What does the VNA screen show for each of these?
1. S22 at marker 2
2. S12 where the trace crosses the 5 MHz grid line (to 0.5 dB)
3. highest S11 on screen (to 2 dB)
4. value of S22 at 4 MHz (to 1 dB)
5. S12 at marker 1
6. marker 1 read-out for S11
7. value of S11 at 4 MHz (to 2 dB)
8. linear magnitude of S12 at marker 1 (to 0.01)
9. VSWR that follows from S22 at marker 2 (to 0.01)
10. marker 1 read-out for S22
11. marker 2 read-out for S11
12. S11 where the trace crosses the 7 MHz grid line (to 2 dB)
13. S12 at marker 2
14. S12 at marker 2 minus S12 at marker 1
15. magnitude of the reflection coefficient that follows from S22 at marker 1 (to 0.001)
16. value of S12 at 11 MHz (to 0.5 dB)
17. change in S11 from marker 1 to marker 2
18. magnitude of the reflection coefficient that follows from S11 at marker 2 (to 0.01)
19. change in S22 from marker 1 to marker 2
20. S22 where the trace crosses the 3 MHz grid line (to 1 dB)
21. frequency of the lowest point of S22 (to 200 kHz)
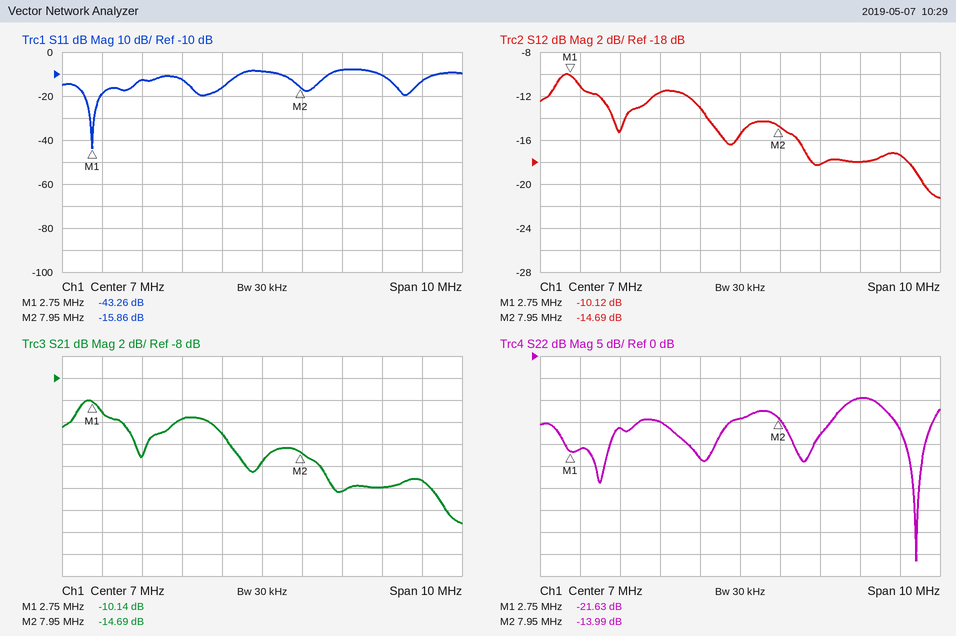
-13.99 dB
-11.5 dB
-8 dB
-16 dB
-10.12 dB
-43.26 dB
-12 dB
0.31
1.50
-21.63 dB
-15.86 dB
-8 dB
-14.69 dB
-4.57 dB
0.083
-17.5 dB
27.40 dB
0.16
7.64 dB
-21 dB
11.4 MHz
